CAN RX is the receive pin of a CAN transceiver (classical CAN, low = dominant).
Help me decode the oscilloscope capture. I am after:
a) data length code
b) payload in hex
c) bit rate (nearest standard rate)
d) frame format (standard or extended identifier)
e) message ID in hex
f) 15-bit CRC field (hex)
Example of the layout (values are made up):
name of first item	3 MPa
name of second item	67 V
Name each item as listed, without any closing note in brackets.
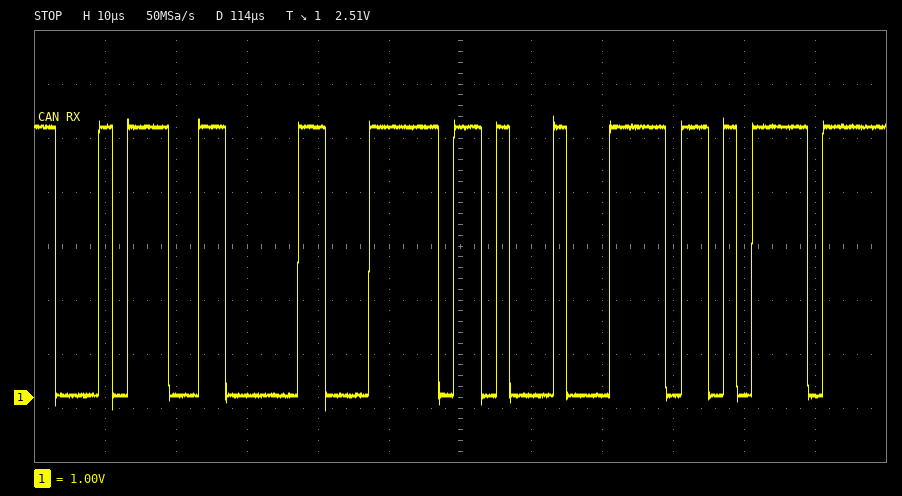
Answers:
data length code	2
payload in hex	3F A2
bit rate	500 kbit/s
frame format	standard
message ID in hex	0x173
15-bit CRC field	0x1ED7
